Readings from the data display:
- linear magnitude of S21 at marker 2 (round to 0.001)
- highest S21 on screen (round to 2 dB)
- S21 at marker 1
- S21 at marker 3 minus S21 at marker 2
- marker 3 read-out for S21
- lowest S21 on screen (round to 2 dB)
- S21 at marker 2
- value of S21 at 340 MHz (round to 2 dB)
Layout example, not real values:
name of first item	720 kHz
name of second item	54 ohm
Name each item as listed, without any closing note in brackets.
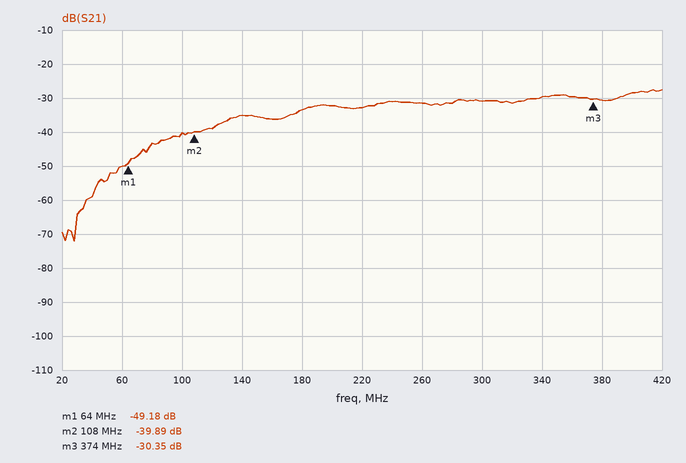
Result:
linear magnitude of S21 at marker 2	0.010
highest S21 on screen	-28 dB
S21 at marker 1	-49.18 dB
S21 at marker 3 minus S21 at marker 2	9.54 dB
marker 3 read-out for S21	-30.35 dB
lowest S21 on screen	-72 dB
S21 at marker 2	-39.89 dB
value of S21 at 340 MHz	-30 dB
